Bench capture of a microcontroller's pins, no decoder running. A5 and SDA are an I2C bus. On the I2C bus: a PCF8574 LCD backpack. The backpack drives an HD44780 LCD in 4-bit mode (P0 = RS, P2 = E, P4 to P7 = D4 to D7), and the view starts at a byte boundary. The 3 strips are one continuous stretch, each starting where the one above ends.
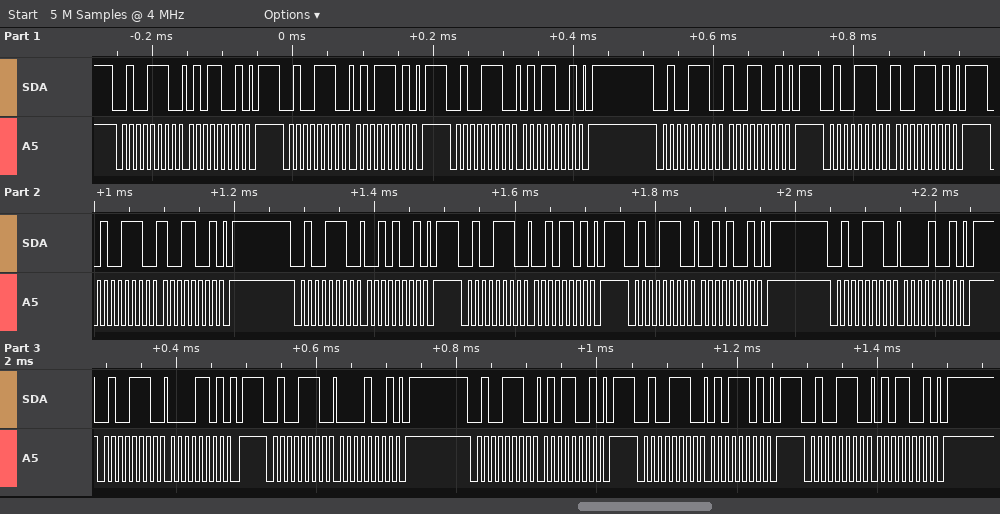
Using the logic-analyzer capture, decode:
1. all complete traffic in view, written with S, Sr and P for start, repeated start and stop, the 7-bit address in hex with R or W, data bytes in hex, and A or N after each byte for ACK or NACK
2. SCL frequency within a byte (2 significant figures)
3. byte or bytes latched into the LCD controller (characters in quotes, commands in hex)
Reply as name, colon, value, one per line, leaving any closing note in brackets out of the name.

all complete traffic in view, written with S, Sr and P for start, repeated start and stop, the 7-bit address in hex with R or W, data bytes in hex, and A or N after each byte for ACK or NACK: S 27W A 59 A P S 27W A 5D A P S 27W A 59 A P S 27W A 99 A P S 27W A 9D A P S 27W A 99 A P S 27W A 29 A P S 27W A 2D A P S 27W A 29 A P S 27W A 09 A P S 27W A 0D A P S 27W A 09 A P S 27W A 59 A P S 27W A 5D A P S 27W A 59 A P
SCL frequency within a byte: 100 kHz
byte or bytes latched into the LCD controller: 'Y' ' '
